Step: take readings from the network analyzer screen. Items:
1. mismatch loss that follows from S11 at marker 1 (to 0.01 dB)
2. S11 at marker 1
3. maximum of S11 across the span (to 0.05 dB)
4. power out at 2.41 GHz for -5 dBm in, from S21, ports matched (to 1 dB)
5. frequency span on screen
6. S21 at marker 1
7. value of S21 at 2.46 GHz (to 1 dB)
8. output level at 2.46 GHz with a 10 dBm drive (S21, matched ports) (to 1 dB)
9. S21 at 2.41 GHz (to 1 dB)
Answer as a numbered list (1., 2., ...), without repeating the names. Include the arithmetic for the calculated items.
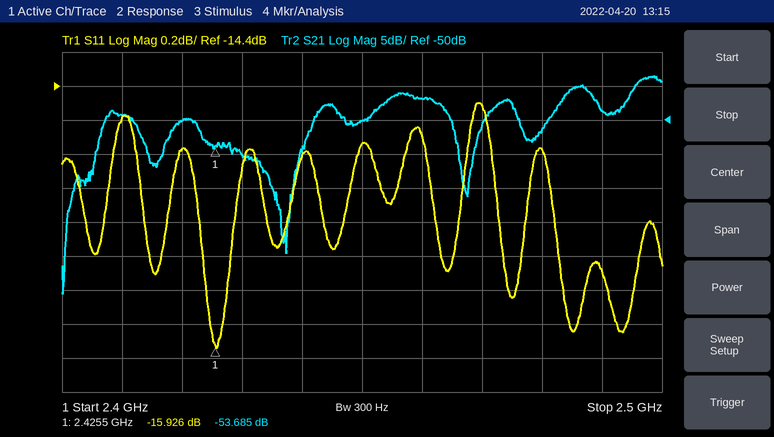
1. −10 log10(1 − 10^(-15.926/10)) ≈ 0.11 dB
2. -15.926 dB
3. -14.50 dB
4. -5 dBm + (-49 dB) = -54 dBm
5. 100 MHz
6. -53.685 dB
7. -47 dB
8. 10 dBm + (-47 dB) = -37 dBm
9. -49 dB
